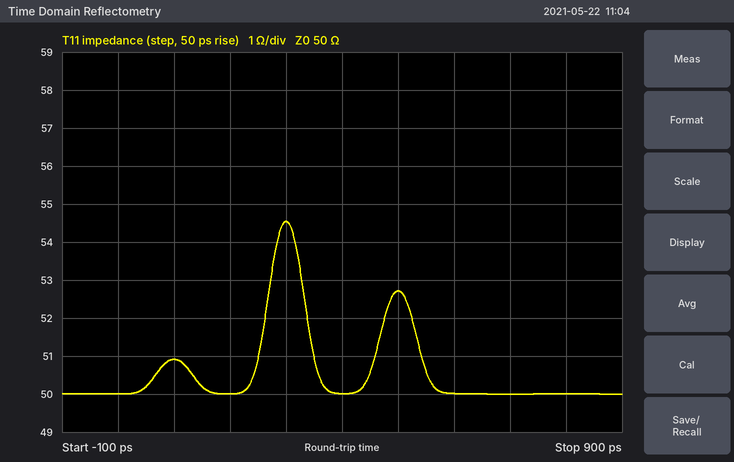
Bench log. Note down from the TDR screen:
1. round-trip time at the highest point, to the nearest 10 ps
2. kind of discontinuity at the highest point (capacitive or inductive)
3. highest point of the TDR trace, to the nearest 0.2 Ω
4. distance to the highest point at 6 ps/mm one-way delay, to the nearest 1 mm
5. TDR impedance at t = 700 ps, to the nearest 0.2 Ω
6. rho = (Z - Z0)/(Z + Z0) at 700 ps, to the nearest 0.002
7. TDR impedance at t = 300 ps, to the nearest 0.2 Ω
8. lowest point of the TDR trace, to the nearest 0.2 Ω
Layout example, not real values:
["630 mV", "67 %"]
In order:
["300 ps", "inductive", "54.6 Ω", "25 mm", "50.0 Ω", "0.000", "54.6 Ω", "50.0 Ω"]
